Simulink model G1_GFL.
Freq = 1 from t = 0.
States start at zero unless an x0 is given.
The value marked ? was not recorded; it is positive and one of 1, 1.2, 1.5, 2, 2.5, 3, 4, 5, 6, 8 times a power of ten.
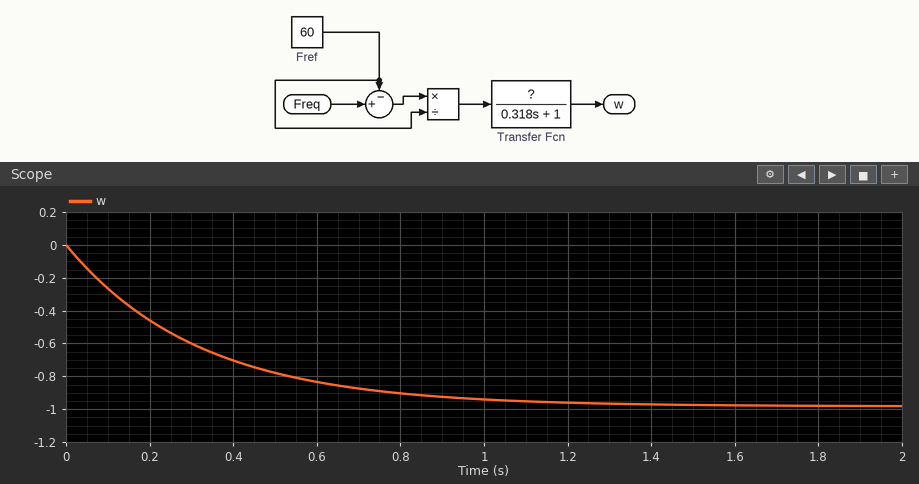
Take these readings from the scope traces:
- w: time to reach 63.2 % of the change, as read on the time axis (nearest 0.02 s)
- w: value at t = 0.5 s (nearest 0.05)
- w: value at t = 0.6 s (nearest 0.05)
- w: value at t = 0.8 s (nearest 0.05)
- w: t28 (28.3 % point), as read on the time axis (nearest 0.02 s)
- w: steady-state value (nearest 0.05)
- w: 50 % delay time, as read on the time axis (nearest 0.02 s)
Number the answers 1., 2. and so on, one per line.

1. 0.32 s
2. -0.80
3. -0.85
4. -0.90
5. 0.10 s
6. -1.00
7. 0.22 s
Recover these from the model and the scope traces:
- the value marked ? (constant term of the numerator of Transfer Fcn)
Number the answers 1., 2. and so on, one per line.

1. 1
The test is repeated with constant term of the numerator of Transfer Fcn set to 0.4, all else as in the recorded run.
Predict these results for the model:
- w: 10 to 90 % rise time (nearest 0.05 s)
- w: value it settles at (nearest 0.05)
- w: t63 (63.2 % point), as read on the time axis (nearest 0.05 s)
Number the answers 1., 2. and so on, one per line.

1. 0.70 s
2. -0.40
3. 0.30 s
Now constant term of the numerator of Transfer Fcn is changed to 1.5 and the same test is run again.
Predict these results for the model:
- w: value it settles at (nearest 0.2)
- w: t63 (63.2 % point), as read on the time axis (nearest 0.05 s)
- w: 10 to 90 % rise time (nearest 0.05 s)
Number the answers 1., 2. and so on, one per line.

1. -1.4
2. 0.30 s
3. 0.70 s
